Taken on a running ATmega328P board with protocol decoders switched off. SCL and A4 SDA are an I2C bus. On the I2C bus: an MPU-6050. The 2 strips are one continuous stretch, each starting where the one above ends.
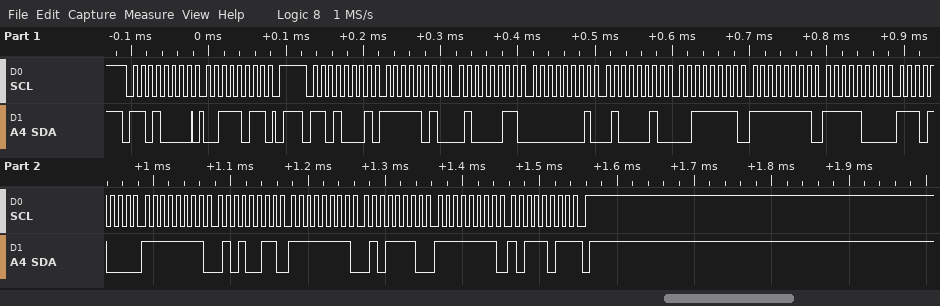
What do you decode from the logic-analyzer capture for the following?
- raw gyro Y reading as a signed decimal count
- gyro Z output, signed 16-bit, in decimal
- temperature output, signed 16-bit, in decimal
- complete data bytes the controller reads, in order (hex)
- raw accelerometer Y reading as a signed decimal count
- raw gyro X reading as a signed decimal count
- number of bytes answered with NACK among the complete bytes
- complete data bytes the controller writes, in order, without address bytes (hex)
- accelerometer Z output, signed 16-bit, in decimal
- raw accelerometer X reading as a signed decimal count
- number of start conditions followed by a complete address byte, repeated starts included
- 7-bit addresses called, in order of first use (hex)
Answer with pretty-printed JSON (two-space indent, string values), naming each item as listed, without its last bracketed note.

{
  "raw gyro Y reading as a signed decimal count": "-162",
  "gyro Z output, signed 16-bit, in decimal": "-69",
  "temperature output, signed 16-bit, in decimal": "-1816",
  "complete data bytes the controller reads, in order": "FA 43 01 42 3F FF F8 E8 FF 53 FF 5E FF BB",
  "raw accelerometer Y reading as a signed decimal count": "322",
  "raw gyro X reading as a signed decimal count": "-173",
  "number of bytes answered with NACK among the complete bytes": "1",
  "complete data bytes the controller writes, in order, without address bytes": "3B",
  "accelerometer Z output, signed 16-bit, in decimal": "16383",
  "raw accelerometer X reading as a signed decimal count": "-1469",
  "number of start conditions followed by a complete address byte, repeated starts included": "2",
  "7-bit addresses called, in order of first use": "0x68"
}
